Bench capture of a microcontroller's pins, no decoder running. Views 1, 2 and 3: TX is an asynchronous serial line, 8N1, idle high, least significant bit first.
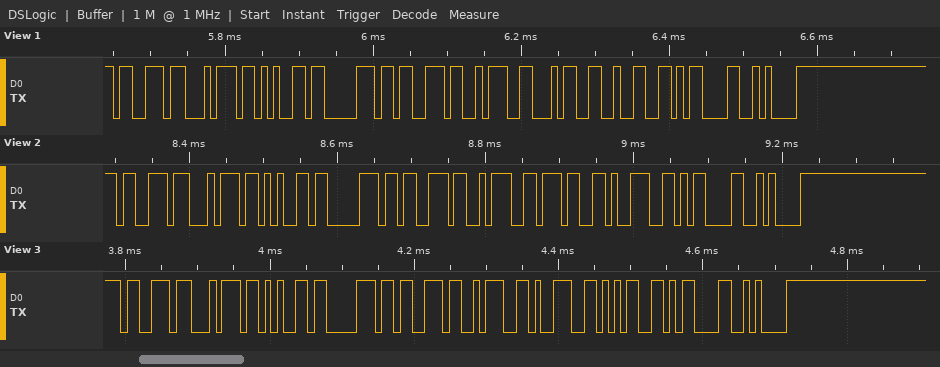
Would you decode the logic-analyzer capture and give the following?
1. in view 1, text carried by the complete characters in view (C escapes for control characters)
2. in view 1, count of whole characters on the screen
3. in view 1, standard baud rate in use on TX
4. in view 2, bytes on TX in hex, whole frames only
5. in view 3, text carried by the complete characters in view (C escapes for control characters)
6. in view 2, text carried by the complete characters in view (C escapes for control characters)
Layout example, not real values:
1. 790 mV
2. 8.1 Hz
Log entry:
1. "steps:42\r\n"
2. 10
3. 115200 baud
4. 73 74 65 70 73 3A 37 39 0D 0A
5. "steps:95\r\n"
6. "steps:79\r\n"
